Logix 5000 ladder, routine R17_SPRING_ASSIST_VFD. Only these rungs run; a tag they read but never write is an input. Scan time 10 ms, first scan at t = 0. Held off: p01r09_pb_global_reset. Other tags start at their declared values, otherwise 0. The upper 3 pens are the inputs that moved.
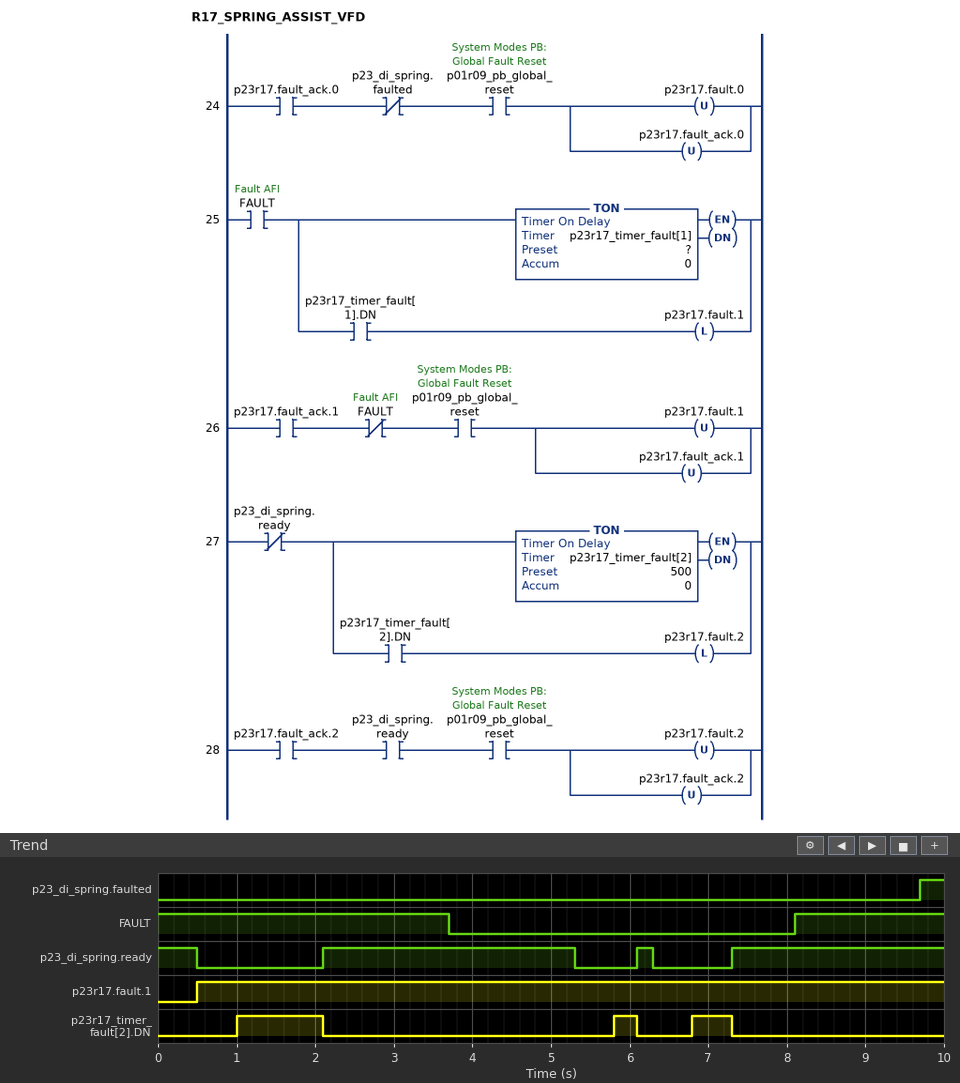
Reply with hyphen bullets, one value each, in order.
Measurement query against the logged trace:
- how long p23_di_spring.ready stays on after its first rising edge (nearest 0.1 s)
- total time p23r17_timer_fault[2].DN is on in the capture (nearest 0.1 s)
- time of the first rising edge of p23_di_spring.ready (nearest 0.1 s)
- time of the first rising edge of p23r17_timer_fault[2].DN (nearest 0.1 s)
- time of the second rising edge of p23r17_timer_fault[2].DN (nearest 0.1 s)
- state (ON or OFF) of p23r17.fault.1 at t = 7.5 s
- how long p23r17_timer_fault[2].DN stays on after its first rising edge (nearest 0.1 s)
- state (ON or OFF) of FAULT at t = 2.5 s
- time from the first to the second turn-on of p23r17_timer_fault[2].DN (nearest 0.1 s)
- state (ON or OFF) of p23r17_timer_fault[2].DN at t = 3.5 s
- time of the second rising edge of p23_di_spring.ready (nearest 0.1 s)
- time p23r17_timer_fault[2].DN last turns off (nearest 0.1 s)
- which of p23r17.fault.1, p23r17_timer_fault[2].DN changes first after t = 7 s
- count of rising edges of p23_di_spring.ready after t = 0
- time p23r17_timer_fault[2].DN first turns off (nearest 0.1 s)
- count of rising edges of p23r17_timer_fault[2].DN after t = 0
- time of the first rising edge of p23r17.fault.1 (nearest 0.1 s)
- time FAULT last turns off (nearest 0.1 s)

- 3.2 s
- 1.9 s
- 2.1 s
- 1.0 s
- 5.8 s
- ON
- 1.1 s
- ON
- 4.8 s
- OFF
- 6.1 s
- 7.3 s
- p23r17_timer_fault[2].DN
- 3
- 2.1 s
- 3
- 0.5 s
- 3.7 s
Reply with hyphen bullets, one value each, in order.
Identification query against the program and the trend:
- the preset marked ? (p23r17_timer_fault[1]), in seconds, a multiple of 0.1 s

- 0.5 s
